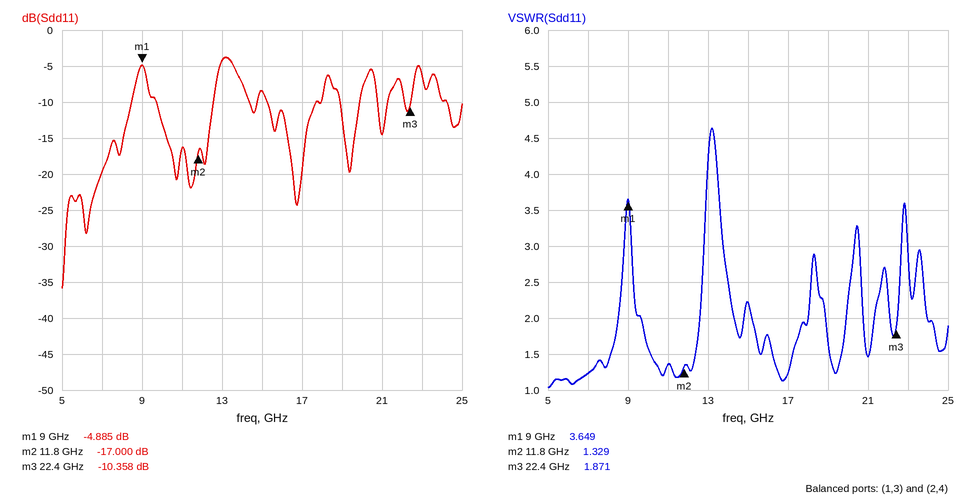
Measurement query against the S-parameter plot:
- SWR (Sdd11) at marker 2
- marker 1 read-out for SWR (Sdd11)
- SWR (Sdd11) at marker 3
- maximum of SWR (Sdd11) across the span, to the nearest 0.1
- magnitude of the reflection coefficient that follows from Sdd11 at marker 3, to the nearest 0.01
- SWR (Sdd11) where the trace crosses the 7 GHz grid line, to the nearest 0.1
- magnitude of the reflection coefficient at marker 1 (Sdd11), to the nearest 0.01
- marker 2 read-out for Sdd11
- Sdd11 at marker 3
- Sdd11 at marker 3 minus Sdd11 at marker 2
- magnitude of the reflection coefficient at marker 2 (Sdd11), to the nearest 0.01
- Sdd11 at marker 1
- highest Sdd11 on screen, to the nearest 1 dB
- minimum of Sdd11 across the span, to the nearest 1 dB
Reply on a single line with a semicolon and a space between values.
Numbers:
1.329; 3.649; 1.871; 4.6; 0.30; 1.2; 0.57; -17.000 dB; -10.358 dB; 6.642 dB; 0.14; -4.885 dB; -4 dB; -36 dB
